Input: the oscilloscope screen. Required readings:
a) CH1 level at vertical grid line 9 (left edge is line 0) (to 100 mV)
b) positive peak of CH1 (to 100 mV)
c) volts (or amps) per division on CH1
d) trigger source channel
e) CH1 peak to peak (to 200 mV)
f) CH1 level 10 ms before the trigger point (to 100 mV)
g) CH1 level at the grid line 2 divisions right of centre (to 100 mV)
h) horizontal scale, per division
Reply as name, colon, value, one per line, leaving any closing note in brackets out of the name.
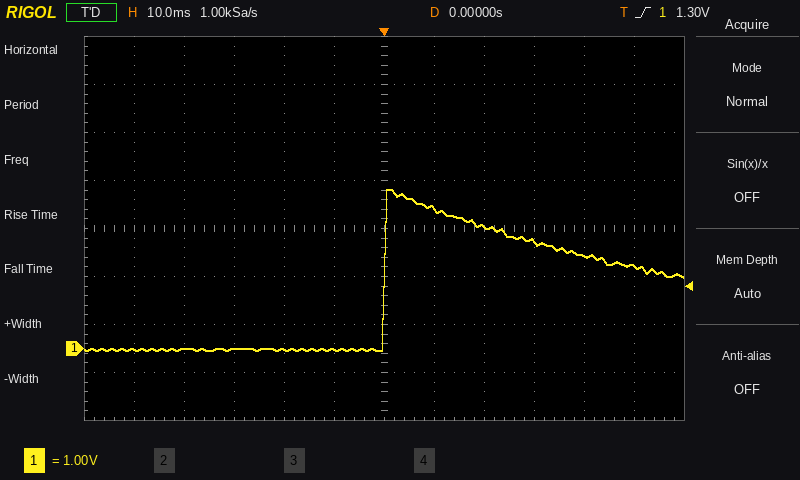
CH1 level at vertical grid line 9 (left edge is line 0): 2.2 V
positive peak of CH1: 3.3 V
volts (or amps) per division on CH1: 1 V
trigger source channel: CH1
CH1 peak to peak: 3.4 V
CH1 level 10 ms before the trigger point: 0.0 V
CH1 level at the grid line 2 divisions right of centre: 2.5 V
horizontal scale, per division: 10 ms
